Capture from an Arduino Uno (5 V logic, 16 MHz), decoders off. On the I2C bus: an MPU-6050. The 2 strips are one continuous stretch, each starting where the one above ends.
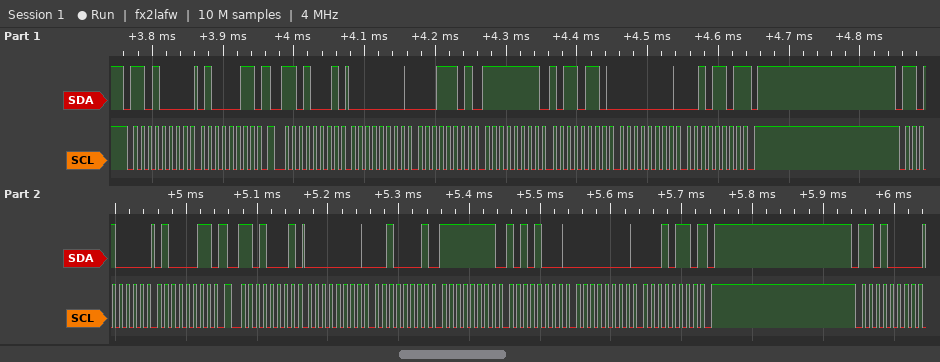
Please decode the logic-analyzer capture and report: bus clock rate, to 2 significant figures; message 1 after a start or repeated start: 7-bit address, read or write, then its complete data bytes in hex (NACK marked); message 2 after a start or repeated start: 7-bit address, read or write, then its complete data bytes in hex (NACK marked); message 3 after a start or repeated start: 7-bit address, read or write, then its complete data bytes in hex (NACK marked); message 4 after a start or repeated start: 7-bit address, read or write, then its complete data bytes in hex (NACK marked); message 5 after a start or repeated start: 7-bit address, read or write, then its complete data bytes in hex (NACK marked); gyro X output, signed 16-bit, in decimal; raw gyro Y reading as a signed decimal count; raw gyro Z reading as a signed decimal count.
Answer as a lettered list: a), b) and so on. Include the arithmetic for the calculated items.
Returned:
a) 100 kHz
b) 0x68 write: 43
c) 0x68 read: 00 1D FF B6 00 2D NACK
d) 0x68 write: 43
e) 0x68 read: 00 21 FF A8 00 16 NACK
f) 0x68 write
g) 0x001D = 29
h) 0xFFB6 = -74
i) 0x002D = 45
